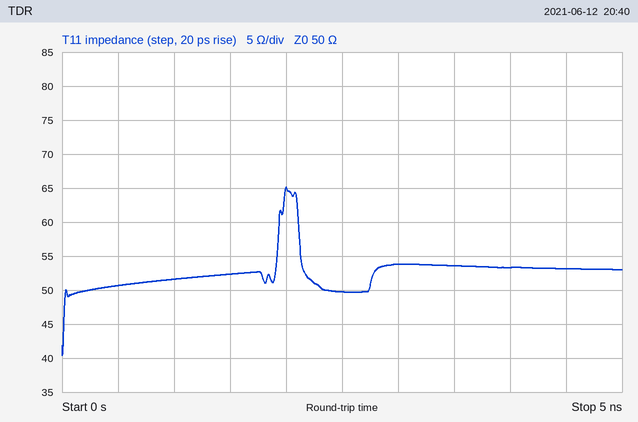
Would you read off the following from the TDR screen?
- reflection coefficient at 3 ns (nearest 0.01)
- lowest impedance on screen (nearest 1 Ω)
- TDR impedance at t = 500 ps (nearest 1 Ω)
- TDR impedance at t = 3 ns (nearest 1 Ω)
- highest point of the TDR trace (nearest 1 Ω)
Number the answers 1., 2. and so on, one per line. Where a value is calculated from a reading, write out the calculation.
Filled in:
1. (54 − 50)/(54 + 50) ≈ +0.04
2. 40 Ω
3. 51 Ω
4. 54 Ω
5. 65 Ω
